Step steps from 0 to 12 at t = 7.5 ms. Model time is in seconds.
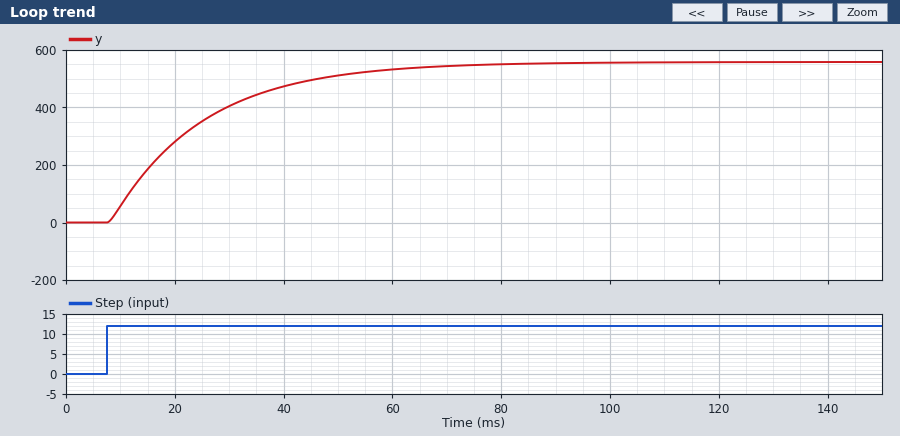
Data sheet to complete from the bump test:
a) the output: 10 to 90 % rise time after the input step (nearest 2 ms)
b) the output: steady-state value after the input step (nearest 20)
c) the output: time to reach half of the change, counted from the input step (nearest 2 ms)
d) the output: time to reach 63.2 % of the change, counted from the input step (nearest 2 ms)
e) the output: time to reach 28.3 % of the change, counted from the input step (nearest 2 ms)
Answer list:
38 ms
560
12 ms
18 ms
6 ms
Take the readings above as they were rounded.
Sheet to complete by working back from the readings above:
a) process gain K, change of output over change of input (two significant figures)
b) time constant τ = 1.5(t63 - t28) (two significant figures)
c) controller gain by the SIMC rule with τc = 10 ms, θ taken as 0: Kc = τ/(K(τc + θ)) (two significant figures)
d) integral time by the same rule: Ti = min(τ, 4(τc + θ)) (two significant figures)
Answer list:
47
18 ms
0.038
18 ms
